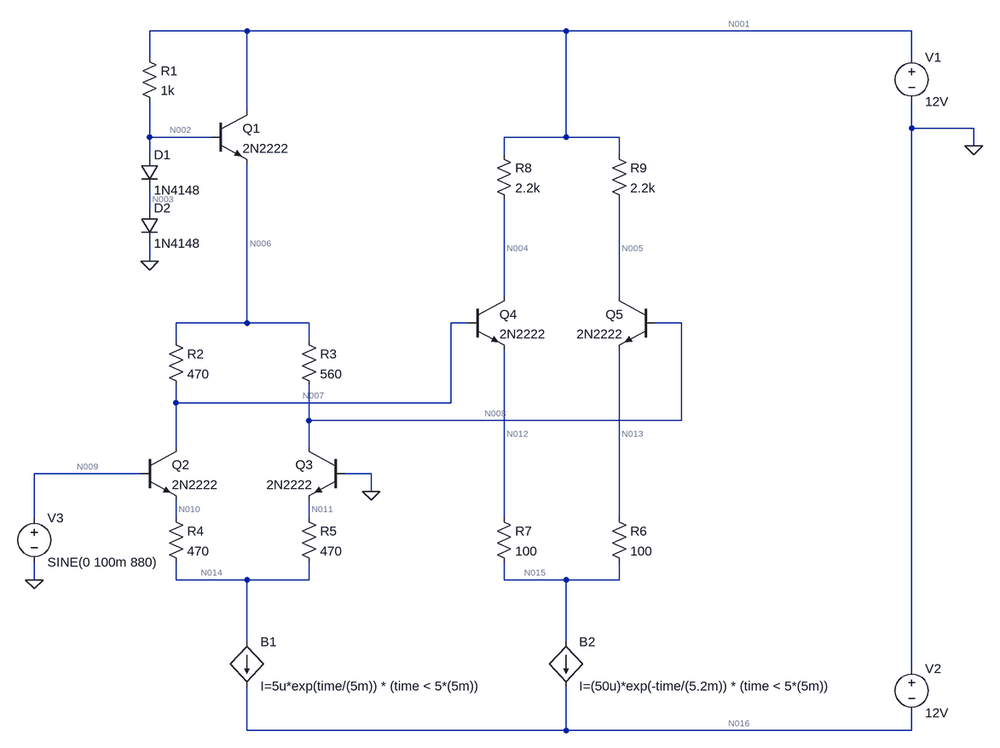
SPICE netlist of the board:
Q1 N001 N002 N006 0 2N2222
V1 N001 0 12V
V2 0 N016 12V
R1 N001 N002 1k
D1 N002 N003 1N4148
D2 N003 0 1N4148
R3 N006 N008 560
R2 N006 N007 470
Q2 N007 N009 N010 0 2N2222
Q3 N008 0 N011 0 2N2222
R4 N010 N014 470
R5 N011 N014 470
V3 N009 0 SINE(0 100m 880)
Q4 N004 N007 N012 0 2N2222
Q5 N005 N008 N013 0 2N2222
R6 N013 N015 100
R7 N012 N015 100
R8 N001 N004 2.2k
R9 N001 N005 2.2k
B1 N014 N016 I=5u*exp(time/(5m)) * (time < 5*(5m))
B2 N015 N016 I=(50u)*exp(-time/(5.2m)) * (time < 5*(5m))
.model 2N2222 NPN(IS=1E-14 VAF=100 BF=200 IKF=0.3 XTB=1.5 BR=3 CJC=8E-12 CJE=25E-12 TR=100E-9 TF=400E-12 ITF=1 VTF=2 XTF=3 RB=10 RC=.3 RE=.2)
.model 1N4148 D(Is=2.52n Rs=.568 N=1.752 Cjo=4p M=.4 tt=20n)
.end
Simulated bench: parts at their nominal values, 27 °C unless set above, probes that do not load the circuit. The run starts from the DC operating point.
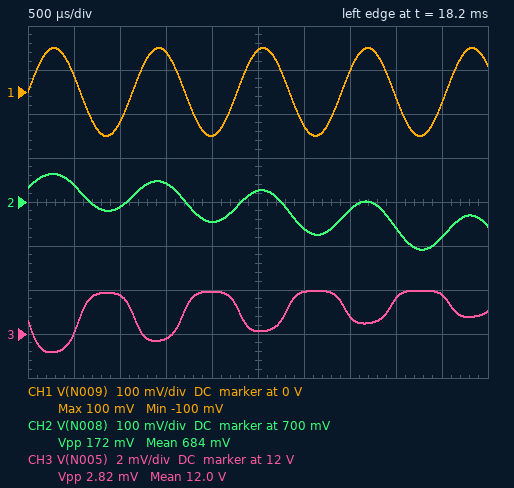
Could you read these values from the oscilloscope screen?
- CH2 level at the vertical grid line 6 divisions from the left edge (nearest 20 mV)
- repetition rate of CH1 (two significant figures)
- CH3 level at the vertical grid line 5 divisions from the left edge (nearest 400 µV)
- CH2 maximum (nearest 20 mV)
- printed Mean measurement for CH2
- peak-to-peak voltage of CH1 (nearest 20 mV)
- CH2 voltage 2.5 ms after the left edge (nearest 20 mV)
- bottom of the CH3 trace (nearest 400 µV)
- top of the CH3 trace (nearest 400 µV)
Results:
640 mV
880 Hz
11.9980 V
760 mV
684 mV
200 mV
720 mV
11.9972 V
12.0000 V
